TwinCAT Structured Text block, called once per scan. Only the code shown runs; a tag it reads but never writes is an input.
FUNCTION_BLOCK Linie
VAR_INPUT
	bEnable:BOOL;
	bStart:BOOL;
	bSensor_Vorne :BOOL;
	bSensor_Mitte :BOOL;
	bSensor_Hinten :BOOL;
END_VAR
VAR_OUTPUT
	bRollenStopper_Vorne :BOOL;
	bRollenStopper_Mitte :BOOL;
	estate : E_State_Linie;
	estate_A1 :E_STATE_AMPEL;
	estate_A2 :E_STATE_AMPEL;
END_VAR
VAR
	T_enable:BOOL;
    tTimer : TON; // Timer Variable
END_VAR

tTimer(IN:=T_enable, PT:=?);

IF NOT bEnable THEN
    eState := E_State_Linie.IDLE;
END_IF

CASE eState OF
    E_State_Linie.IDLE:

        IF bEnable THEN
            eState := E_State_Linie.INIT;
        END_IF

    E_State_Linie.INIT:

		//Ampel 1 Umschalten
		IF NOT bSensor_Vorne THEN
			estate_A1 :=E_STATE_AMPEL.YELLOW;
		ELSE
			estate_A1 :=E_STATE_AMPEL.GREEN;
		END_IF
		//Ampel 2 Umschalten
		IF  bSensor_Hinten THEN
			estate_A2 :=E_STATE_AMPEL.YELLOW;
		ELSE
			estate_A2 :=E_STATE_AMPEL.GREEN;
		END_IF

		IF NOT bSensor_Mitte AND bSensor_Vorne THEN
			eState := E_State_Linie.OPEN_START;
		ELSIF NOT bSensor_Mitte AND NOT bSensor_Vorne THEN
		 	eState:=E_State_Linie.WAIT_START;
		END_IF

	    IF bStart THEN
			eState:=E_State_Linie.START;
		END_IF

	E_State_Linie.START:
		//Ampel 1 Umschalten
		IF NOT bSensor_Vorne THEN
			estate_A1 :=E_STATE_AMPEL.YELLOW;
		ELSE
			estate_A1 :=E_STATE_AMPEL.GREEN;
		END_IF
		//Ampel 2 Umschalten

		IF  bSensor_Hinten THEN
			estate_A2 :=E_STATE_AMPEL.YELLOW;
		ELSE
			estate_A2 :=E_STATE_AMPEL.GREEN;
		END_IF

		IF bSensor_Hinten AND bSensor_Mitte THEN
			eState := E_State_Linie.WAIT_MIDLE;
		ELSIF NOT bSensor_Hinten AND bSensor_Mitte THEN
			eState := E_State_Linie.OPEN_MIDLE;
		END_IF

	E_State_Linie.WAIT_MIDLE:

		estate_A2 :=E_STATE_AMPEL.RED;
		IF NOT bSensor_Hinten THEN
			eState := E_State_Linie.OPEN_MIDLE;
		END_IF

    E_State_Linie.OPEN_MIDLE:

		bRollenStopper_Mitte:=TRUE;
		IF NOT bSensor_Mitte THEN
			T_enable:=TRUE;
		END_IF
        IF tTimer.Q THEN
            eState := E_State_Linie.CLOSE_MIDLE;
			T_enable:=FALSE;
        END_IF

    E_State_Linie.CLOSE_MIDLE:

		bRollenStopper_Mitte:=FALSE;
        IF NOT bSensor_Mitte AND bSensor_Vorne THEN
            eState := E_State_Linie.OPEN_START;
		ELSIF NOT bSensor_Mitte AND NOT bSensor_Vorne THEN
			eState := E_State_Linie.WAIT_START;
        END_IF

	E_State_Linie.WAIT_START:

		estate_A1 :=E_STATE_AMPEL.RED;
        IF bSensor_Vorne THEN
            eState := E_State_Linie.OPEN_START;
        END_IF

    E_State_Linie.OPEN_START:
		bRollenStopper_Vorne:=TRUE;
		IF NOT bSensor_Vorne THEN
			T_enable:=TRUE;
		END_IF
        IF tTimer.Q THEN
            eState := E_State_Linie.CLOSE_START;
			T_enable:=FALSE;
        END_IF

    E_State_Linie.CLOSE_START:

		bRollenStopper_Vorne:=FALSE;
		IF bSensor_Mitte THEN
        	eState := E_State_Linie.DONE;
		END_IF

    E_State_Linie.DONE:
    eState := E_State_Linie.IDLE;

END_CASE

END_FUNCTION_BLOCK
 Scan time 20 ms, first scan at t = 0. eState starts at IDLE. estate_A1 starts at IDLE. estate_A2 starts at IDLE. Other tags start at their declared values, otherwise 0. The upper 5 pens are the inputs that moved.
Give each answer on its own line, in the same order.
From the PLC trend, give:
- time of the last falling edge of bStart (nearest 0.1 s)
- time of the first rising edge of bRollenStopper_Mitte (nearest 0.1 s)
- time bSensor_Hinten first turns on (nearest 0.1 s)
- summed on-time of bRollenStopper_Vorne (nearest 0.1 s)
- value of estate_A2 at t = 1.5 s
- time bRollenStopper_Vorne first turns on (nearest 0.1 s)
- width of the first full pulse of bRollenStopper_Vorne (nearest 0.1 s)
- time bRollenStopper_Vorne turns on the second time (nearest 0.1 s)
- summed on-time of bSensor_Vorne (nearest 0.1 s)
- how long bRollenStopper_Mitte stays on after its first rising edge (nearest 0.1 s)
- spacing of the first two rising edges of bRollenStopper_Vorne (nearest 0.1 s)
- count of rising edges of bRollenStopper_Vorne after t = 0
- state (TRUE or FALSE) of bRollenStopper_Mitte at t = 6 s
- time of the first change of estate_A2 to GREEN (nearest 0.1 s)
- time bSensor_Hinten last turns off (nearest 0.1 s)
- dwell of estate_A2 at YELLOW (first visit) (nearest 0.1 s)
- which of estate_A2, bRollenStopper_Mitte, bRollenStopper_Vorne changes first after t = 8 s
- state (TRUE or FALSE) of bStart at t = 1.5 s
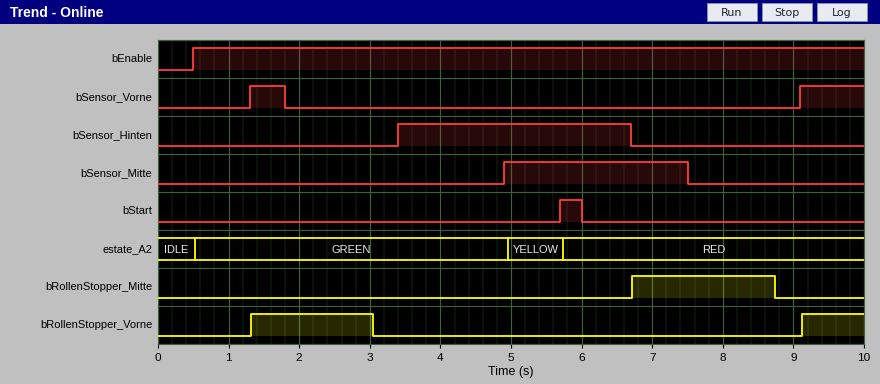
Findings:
6.0 s
6.7 s
3.4 s
2.6 s
GREEN
1.3 s
1.7 s
9.1 s
1.4 s
2.0 s
7.8 s
2
FALSE
0.5 s
6.7 s
0.8 s
bRollenStopper_Mitte
FALSE
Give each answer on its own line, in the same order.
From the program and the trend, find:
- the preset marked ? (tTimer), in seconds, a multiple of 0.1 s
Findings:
1.2 s
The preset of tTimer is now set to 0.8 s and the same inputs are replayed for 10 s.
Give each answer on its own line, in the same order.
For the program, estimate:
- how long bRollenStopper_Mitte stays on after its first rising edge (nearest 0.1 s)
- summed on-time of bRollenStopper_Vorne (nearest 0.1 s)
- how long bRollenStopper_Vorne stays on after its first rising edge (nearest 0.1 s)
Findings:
1.6 s
2.2 s
1.3 s
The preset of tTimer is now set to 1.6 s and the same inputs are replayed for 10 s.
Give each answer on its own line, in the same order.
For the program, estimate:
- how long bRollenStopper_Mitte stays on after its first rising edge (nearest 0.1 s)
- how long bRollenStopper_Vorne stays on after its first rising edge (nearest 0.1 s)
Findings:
2.4 s
2.1 s
